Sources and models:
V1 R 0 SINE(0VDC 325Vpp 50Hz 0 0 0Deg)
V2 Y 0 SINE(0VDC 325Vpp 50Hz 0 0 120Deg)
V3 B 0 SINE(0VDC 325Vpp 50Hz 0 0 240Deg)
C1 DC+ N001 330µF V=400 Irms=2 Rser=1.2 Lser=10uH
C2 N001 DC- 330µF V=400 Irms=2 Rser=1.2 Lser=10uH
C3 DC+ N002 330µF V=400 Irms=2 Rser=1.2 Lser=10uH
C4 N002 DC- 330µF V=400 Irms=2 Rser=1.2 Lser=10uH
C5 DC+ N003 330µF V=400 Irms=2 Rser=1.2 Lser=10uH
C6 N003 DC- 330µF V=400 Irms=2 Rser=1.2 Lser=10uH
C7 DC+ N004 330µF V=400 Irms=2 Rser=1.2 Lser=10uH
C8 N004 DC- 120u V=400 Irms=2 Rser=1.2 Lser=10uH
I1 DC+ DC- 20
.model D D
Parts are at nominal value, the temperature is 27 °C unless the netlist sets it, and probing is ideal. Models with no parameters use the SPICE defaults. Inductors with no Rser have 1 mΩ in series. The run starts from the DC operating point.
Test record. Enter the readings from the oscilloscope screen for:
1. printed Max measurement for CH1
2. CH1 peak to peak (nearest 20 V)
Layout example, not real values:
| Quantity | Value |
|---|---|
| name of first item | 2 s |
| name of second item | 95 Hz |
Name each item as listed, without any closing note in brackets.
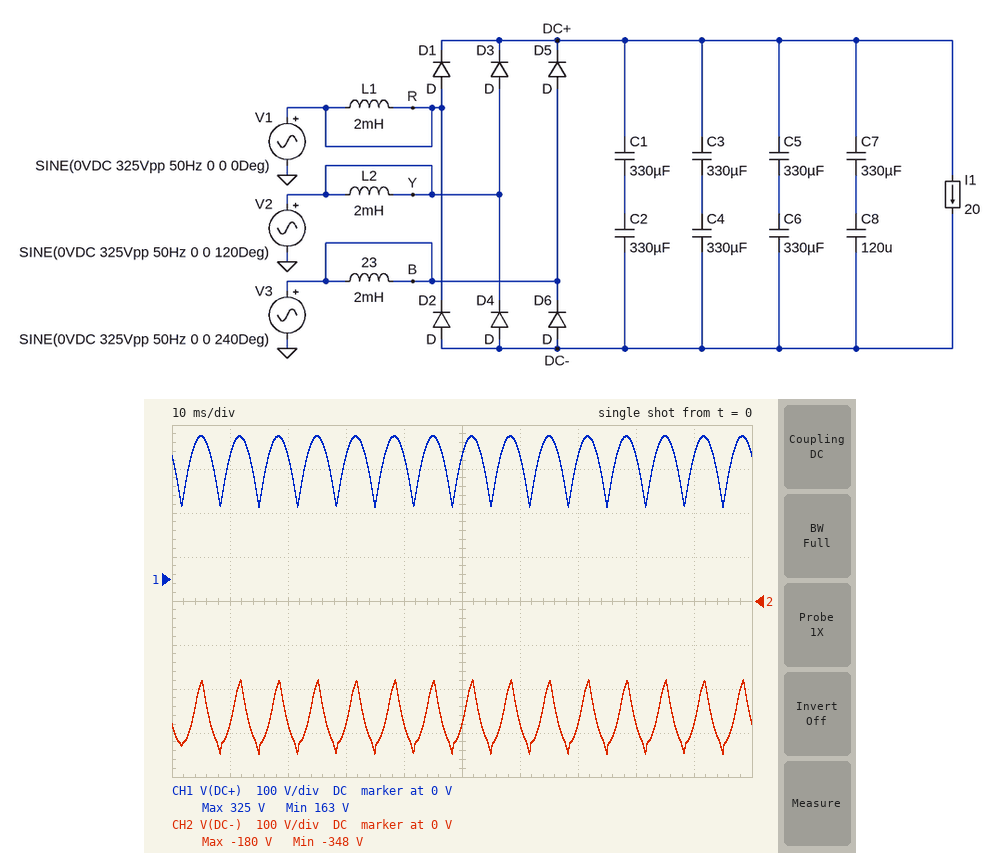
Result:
| Quantity | Value |
|---|---|
| printed Max measurement for CH1 | 325 V |
| CH1 peak to peak | 160 V |
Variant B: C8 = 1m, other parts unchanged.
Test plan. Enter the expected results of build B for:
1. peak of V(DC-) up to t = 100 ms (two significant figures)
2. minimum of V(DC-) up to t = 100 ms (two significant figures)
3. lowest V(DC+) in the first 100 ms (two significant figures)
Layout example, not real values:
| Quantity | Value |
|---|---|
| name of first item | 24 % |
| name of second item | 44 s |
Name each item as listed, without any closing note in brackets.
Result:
| Quantity | Value |
|---|---|
| peak of V(DC-) up to t = 100 ms | -190 V |
| minimum of V(DC-) up to t = 100 ms | -340 V |
| lowest V(DC+) in the first 100 ms | 160 V |
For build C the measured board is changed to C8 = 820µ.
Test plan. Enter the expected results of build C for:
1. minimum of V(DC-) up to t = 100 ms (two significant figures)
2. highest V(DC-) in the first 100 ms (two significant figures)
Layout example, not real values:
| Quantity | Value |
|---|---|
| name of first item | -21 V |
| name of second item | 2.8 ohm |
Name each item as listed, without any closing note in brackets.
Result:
| Quantity | Value |
|---|---|
| minimum of V(DC-) up to t = 100 ms | -340 V |
| highest V(DC-) in the first 100 ms | -190 V |
